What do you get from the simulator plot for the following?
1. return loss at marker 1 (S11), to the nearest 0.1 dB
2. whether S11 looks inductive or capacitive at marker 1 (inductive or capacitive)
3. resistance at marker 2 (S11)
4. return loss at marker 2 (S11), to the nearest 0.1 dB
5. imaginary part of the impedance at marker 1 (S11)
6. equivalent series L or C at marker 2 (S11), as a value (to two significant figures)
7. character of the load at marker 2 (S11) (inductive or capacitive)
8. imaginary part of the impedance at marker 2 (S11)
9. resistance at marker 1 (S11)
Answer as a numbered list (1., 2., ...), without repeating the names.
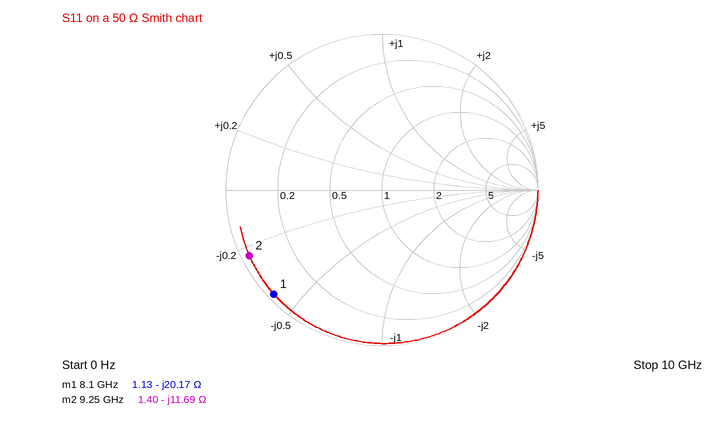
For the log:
1. 0.3 dB
2. capacitive
3. 1.40 Ω
4. 0.5 dB
5. -20.17 Ω
6. 1.5 pF
7. capacitive
8. -11.69 Ω
9. 1.13 Ω
